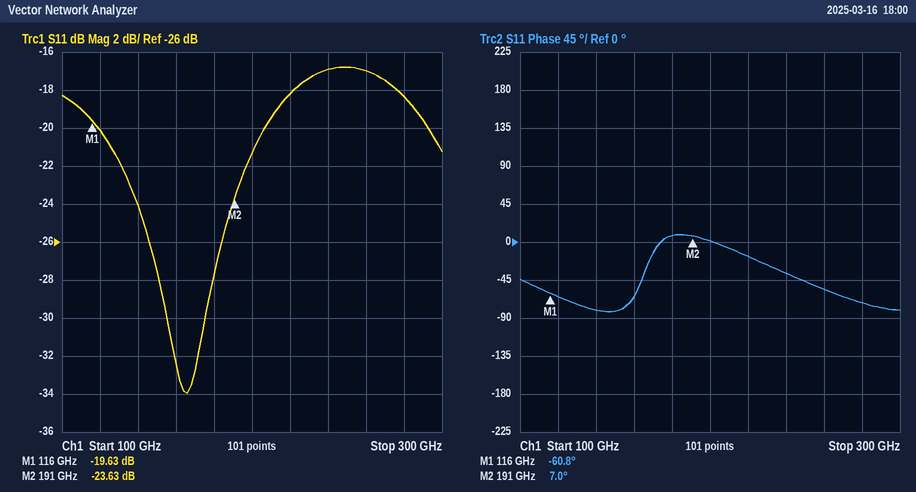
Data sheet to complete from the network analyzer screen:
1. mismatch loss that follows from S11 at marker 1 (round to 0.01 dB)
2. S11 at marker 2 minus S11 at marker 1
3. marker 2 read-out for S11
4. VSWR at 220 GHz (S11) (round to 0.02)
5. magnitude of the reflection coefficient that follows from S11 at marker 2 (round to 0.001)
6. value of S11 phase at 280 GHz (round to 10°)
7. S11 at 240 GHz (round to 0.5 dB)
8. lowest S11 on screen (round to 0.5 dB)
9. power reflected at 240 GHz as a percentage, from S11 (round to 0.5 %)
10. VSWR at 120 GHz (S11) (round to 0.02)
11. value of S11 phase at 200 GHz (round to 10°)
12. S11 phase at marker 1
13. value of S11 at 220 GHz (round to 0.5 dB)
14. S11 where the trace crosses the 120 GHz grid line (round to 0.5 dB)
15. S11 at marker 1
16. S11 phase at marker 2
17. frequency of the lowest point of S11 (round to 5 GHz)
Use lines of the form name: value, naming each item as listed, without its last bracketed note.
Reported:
mismatch loss that follows from S11 at marker 1: 0.05 dB
S11 at marker 2 minus S11 at marker 1: -4.00 dB
marker 2 read-out for S11: -23.63 dB
VSWR at 220 GHz (S11): 1.28
magnitude of the reflection coefficient that follows from S11 at marker 2: 0.066
value of S11 phase at 280 GHz: -70°
S11 at 240 GHz: -17.0 dB
lowest S11 on screen: -34.0 dB
power reflected at 240 GHz as a percentage, from S11: 2.0 %
VSWR at 120 GHz (S11): 1.22
value of S11 phase at 200 GHz: 0°
S11 phase at marker 1: -60.8°
value of S11 at 220 GHz: -18.0 dB
S11 where the trace crosses the 120 GHz grid line: -20.0 dB
S11 at marker 1: -19.63 dB
S11 phase at marker 2: 7.0°
frequency of the lowest point of S11: 165 GHz
